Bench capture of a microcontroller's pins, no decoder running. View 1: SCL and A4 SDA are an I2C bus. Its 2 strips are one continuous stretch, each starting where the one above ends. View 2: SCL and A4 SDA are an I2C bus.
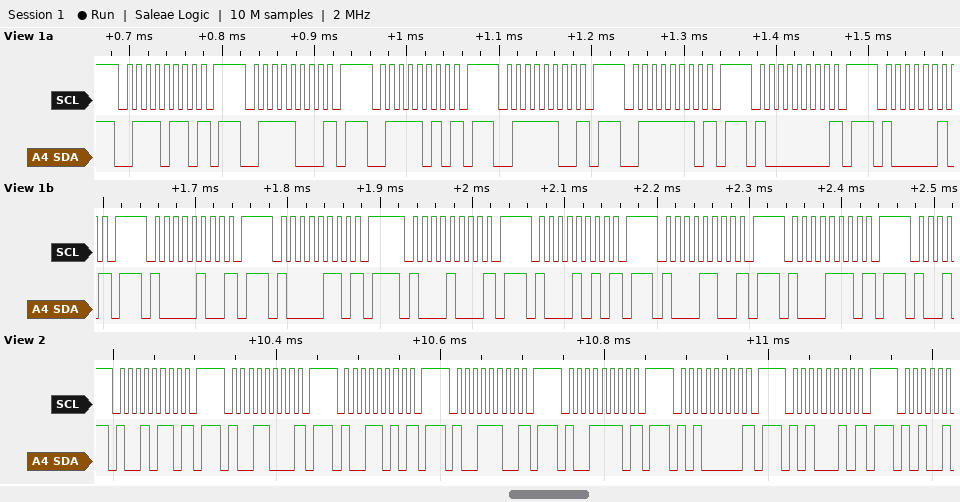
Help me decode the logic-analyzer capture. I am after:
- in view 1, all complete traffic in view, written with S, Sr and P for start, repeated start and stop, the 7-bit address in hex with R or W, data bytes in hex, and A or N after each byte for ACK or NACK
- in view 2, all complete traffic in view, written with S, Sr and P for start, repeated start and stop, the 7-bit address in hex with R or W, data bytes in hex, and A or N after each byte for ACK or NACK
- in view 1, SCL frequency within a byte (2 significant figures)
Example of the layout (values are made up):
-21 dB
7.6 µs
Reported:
S 3BW N P S 3CW N P S 3DW N P S 3EW N P S 3FW N P S 40W N P S 41W N P S 42W N P S 43W N P S 44W N P S 45W N P S 46W N P S 47W N P
S 4BW N P S 4CW N P S 4DW N P S 4EW N P S 4FW N P S 50W N P S 51W N P
100 kHz
